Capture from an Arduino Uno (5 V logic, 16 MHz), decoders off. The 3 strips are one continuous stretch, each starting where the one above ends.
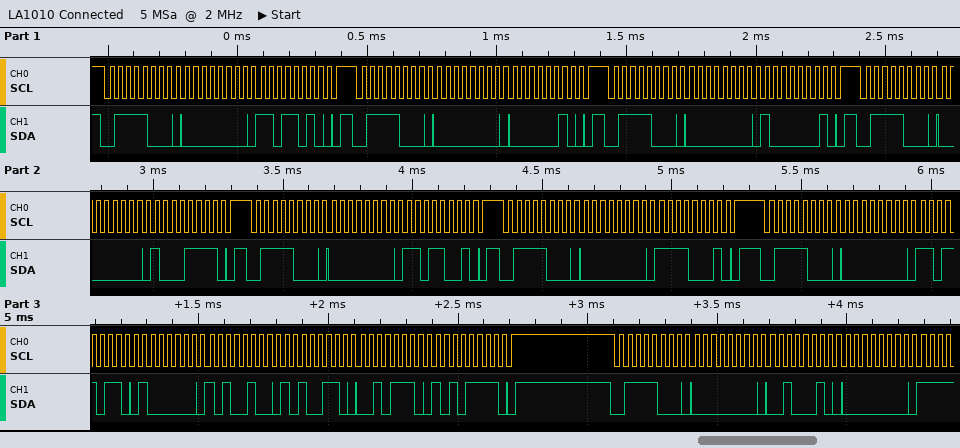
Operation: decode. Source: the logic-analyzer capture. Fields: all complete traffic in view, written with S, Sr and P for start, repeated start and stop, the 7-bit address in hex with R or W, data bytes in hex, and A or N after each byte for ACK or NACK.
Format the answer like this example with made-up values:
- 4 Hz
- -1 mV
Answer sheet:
- S 3CW A 00 A DA A P S 3CW A 00 A 02 A P S 3CW A 00 A 81 A P S 3CW A 00 A 8F A P S 3CW A 00 A D9 A P S 3CW A 00 A F1 A P S 3CW A 00 A DB A 40 A A4 A A6 A 2E A AF A P S 3CW A 00 A 22 A 00 A
